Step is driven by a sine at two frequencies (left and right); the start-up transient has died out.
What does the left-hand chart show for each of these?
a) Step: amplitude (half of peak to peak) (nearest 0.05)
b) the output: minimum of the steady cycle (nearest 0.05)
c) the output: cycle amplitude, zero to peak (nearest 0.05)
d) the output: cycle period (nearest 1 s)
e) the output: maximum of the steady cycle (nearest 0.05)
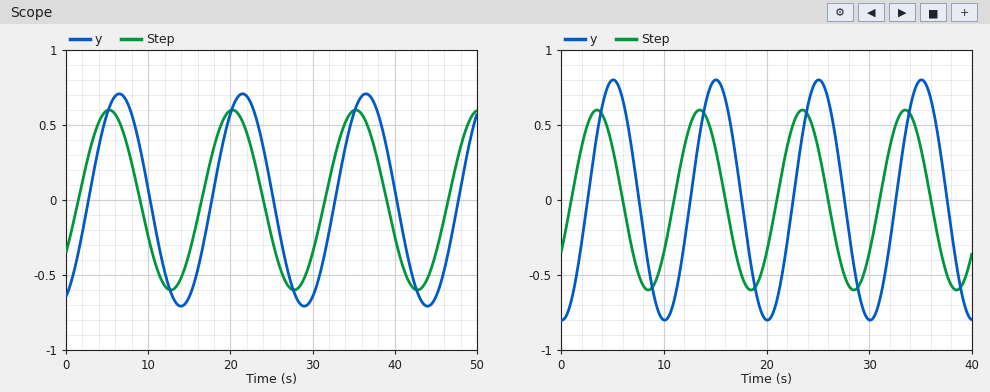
0.60
-0.70
0.70
15 s
0.70
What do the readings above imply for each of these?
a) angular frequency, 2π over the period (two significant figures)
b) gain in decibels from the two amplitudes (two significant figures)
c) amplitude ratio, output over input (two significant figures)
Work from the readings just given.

0.42 rad/s
1.3 dB
1.2
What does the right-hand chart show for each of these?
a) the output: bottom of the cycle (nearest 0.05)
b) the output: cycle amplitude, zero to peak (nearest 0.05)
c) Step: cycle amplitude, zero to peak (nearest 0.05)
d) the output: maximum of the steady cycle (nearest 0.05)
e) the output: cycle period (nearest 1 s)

-0.80
0.80
0.60
0.80
10 s
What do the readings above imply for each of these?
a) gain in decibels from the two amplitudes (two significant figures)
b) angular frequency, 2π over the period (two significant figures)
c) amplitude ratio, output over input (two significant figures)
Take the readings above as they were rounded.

2.5 dB
0.63 rad/s
1.3
